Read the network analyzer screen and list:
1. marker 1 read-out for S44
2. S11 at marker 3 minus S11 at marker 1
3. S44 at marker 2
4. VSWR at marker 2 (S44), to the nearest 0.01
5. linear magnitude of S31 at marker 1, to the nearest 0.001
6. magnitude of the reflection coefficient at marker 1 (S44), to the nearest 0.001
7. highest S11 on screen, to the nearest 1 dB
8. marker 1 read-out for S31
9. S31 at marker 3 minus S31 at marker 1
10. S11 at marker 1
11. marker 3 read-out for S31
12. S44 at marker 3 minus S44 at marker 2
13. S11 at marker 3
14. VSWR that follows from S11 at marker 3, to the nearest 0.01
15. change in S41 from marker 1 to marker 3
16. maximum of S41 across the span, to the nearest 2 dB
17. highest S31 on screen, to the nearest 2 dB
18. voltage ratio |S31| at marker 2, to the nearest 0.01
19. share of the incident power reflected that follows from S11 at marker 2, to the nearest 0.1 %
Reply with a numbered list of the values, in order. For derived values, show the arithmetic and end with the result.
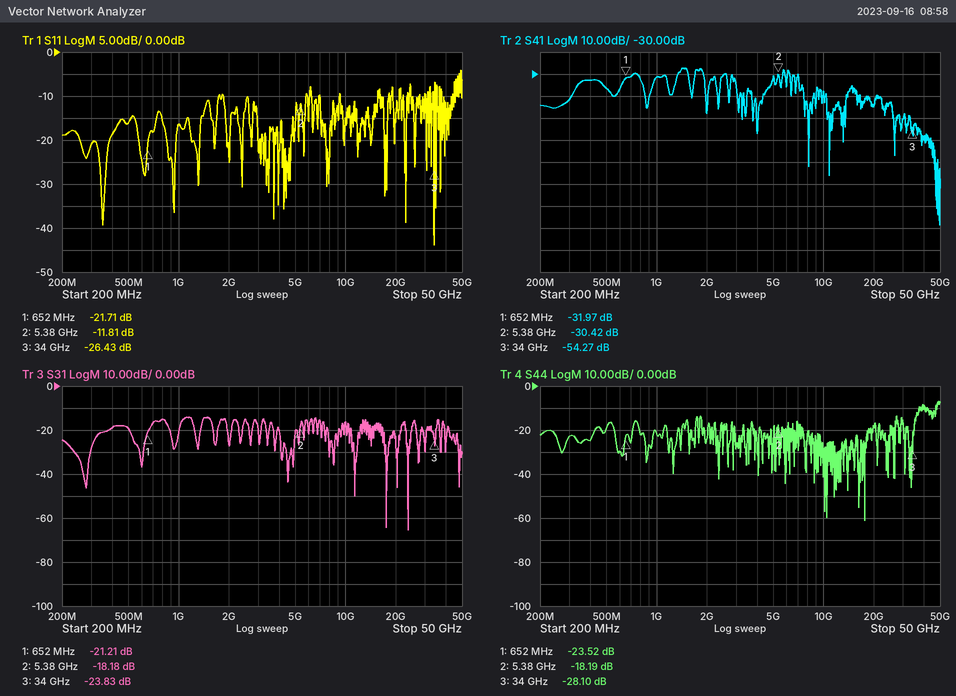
1. -23.52 dB
2. -26.43 − (-21.71) = -4.72 dB
3. -18.19 dB
4. (1 + 0.1232)/(1 − 0.1232) ≈ 1.28
5. 10^(-21.21/20) ≈ 0.087
6. 10^(-23.52/20) ≈ 0.067
7. -4 dB
8. -21.21 dB
9. -23.83 − (-21.21) = -2.62 dB
10. -21.71 dB
11. -23.83 dB
12. -28.1 − (-18.19) = -9.91 dB
13. -26.43 dB
14. (1 + 0.0477)/(1 − 0.0477) ≈ 1.10
15. -54.27 − (-31.97) = -22.30 dB
16. -28 dB
17. -14 dB
18. 10^(-18.18/20) ≈ 0.12
19. 10^(-11.81/10) ≈ 6.6 %
